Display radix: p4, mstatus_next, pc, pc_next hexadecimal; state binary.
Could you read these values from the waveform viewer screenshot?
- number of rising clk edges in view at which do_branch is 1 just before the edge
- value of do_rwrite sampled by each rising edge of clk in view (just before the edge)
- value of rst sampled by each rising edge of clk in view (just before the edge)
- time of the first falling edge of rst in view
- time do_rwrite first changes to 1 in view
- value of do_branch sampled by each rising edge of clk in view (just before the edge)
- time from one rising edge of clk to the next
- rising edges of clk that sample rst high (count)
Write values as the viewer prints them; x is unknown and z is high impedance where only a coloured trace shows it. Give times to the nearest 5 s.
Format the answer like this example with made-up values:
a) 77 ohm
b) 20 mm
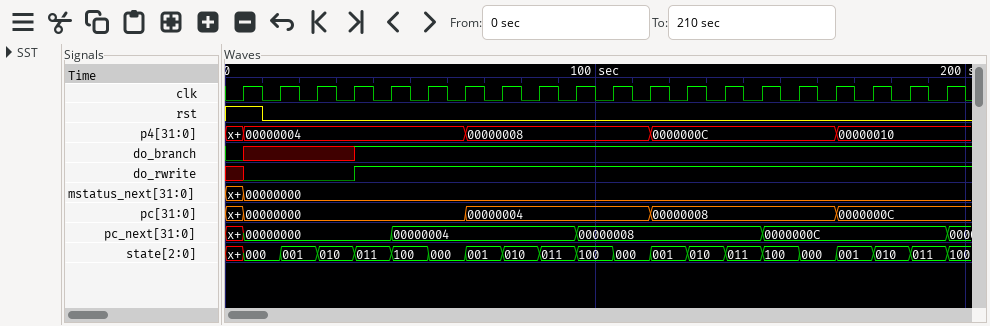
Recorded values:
a) 16
b) x 0 0 0 1 1 1 1 1 1 1 1 1 1 1 1 1 1 1 1
c) 1 0 0 0 0 0 0 0 0 0 0 0 0 0 0 0 0 0 0 0
d) 10 s
e) 35 s
f) 0 x x x 1 1 1 1 1 1 1 1 1 1 1 1 1 1 1 1
g) 10 s
h) 1
